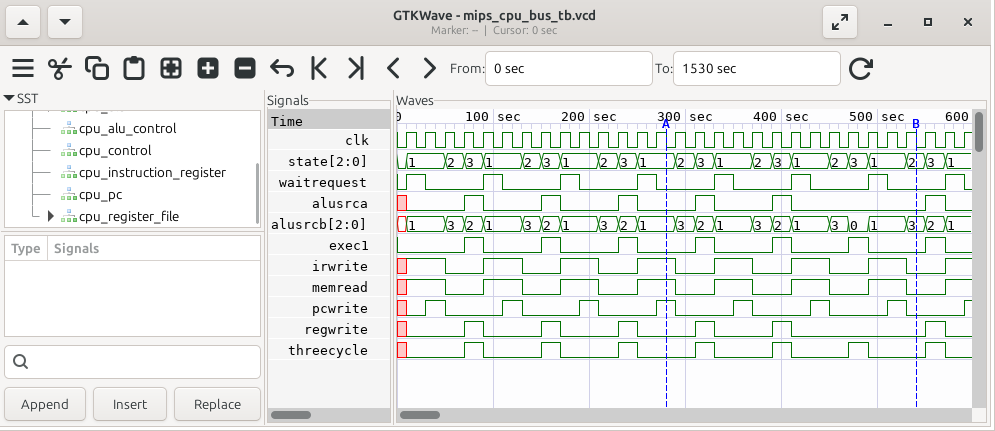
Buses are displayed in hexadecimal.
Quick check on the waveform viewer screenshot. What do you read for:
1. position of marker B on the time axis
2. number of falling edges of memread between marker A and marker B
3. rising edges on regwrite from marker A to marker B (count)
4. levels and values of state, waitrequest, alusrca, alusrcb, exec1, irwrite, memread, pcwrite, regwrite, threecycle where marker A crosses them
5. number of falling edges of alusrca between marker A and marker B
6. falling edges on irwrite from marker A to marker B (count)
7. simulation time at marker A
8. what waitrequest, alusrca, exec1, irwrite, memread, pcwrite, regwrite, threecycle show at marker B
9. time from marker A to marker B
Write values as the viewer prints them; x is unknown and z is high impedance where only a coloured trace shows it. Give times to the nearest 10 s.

540 s
4
2
state=1, waitrequest=0, alusrca=0, alusrcb=1, exec1=0, irwrite=1, memread=1, pcwrite=1, regwrite=0, threecycle=0
2
4
280 s
waitrequest=0, alusrca=0, exec1=0, irwrite=0, memread=0, pcwrite=0, regwrite=0, threecycle=0
260 s
